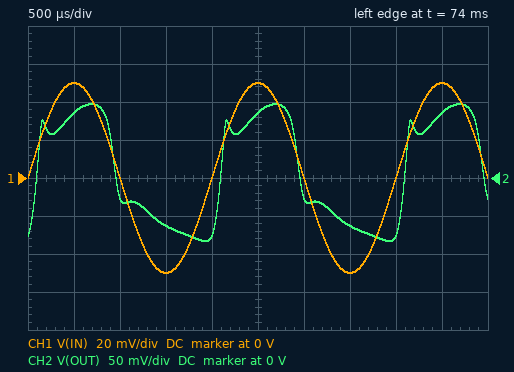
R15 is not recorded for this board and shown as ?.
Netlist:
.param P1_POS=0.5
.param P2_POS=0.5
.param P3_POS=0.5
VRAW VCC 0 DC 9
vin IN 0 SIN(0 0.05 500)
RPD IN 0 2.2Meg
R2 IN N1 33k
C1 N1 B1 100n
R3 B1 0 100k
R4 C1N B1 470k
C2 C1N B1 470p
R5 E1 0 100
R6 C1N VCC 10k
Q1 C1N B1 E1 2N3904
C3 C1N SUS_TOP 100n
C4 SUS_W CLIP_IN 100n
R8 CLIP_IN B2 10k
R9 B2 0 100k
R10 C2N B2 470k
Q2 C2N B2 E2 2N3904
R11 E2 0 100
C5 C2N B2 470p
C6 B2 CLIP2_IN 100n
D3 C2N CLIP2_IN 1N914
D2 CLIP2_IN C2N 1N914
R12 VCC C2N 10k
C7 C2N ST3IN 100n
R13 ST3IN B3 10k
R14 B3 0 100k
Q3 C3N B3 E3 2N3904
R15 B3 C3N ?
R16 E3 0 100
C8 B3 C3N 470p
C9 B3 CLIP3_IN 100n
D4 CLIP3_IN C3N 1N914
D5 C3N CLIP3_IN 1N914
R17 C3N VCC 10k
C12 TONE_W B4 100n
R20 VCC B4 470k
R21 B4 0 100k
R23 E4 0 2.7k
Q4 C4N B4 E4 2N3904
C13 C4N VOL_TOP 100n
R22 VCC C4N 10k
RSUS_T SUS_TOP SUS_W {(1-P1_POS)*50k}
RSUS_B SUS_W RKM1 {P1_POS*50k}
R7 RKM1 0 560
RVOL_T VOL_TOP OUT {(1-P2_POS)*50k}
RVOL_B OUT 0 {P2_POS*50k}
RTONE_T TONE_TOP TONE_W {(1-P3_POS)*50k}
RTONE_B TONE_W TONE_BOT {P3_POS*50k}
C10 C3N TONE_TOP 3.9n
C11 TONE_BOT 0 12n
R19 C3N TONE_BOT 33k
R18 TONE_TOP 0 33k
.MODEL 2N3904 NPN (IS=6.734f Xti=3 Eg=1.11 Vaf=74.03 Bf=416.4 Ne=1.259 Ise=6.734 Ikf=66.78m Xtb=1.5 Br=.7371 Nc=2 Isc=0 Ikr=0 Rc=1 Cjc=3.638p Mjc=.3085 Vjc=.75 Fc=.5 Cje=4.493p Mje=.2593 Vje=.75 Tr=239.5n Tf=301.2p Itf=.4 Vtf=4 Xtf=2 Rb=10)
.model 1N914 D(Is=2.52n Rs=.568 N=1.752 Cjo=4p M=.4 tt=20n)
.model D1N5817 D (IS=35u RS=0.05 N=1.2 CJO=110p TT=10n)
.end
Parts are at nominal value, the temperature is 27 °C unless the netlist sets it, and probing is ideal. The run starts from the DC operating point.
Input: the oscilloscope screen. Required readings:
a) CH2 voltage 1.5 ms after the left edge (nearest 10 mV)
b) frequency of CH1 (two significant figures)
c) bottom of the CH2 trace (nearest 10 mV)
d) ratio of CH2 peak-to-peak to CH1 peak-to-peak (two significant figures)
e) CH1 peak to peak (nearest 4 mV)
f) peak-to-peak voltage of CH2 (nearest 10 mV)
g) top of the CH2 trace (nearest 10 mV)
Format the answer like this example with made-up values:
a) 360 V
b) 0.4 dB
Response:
a) -60 mV
b) 500 Hz
c) -80 mV
d) 1.8
e) 100 mV
f) 180 mV
g) 100 mV
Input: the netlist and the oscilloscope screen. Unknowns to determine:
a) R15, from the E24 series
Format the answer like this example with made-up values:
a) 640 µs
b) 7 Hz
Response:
a) 1.1 MΩ
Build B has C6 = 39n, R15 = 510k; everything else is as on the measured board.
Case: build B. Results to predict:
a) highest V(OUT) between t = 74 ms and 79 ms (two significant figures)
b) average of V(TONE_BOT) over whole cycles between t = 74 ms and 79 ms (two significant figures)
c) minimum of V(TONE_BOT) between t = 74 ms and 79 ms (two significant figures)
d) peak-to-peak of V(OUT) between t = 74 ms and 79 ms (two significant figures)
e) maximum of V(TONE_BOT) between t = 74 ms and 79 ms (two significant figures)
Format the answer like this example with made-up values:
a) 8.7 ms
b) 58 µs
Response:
a) 130 mV
b) 5.0 V
c) 4.8 V
d) 270 mV
e) 5.2 V
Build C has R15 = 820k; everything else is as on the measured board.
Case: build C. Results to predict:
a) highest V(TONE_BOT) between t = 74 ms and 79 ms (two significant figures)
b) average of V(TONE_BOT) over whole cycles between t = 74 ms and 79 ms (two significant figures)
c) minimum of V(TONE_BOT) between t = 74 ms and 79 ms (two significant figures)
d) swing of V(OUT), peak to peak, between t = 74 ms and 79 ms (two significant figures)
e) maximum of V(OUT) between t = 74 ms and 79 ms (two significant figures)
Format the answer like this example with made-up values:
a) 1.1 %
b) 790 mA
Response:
a) 5.7 V
b) 5.5 V
c) 5.3 V
d) 240 mV
e) 120 mV
